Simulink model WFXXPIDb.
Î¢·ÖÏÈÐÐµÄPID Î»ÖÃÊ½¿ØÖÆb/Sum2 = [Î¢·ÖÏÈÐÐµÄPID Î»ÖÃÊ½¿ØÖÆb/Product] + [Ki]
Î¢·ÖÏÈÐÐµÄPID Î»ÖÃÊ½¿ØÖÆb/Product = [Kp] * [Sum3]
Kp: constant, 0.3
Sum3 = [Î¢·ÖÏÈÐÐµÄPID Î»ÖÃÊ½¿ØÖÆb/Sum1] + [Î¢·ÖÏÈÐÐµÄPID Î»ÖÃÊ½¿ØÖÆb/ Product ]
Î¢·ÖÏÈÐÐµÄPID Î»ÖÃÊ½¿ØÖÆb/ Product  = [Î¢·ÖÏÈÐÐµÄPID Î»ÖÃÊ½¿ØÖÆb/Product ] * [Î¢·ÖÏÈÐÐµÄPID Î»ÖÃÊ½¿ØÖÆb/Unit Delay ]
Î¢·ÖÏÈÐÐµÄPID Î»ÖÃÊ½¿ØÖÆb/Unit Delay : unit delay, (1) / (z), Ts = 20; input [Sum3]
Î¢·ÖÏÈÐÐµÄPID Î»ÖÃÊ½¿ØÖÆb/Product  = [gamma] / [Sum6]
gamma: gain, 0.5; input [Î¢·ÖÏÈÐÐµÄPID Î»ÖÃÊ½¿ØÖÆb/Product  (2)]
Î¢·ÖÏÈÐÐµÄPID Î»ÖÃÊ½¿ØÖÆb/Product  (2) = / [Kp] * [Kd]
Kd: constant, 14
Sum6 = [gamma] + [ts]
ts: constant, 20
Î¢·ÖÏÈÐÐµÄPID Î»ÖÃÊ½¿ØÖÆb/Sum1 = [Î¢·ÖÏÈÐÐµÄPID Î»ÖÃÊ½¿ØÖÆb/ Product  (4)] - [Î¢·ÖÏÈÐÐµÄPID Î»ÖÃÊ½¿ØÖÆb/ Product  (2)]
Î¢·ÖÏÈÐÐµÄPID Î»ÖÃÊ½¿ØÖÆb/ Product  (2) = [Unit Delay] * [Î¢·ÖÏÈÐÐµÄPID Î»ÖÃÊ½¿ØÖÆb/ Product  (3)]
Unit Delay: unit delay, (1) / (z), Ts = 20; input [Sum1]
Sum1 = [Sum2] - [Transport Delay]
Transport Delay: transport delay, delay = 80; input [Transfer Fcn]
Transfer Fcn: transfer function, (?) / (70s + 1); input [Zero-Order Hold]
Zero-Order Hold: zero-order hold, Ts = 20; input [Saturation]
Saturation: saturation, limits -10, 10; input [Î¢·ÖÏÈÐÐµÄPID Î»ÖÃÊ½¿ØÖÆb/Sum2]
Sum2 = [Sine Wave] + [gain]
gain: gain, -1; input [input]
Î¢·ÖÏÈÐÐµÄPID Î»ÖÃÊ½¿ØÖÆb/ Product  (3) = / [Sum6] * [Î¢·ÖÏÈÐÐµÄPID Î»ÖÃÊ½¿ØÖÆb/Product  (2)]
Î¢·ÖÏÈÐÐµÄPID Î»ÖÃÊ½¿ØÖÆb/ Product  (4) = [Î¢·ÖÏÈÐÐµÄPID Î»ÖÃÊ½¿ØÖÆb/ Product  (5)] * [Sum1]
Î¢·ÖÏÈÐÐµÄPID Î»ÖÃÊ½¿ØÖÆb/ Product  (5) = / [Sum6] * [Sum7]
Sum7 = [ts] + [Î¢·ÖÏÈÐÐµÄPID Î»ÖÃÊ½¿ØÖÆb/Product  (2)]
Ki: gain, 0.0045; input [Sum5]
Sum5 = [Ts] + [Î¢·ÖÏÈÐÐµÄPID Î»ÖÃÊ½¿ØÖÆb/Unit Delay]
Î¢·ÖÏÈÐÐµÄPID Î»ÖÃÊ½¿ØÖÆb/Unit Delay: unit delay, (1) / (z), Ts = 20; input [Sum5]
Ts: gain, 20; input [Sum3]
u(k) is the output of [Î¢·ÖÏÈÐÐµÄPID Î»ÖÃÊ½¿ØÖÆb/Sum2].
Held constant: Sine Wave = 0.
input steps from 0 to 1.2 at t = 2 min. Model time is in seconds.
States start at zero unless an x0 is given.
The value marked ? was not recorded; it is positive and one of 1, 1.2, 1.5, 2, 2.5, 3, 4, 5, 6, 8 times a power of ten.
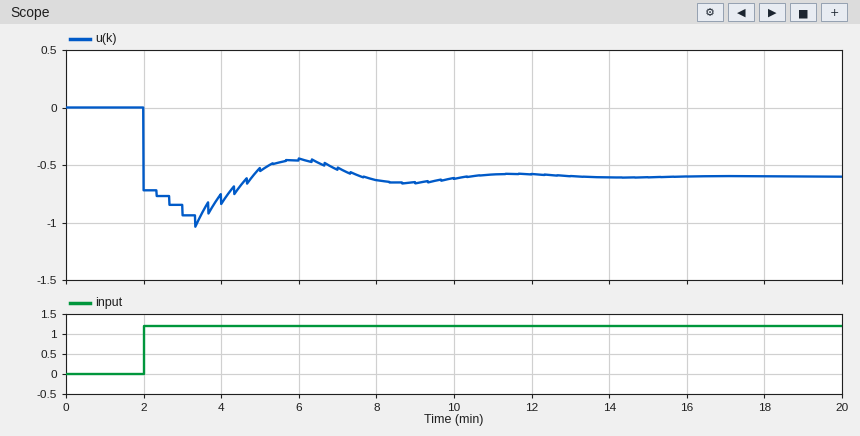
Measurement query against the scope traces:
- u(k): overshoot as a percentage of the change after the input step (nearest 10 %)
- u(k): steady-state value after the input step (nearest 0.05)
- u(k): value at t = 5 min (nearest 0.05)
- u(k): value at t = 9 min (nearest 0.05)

70 %
-0.60
-0.55
-0.65
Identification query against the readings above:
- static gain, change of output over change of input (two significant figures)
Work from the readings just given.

-0.50
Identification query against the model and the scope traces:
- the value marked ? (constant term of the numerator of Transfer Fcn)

2
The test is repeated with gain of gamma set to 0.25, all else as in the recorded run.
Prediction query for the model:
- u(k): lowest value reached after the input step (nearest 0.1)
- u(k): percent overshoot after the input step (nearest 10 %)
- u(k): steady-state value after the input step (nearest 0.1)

-1.1
80 %
-0.6
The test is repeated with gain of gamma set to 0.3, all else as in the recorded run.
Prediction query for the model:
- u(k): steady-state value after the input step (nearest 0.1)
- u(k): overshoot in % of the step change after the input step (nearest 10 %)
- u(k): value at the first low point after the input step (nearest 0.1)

-0.6
80 %
-1.1
